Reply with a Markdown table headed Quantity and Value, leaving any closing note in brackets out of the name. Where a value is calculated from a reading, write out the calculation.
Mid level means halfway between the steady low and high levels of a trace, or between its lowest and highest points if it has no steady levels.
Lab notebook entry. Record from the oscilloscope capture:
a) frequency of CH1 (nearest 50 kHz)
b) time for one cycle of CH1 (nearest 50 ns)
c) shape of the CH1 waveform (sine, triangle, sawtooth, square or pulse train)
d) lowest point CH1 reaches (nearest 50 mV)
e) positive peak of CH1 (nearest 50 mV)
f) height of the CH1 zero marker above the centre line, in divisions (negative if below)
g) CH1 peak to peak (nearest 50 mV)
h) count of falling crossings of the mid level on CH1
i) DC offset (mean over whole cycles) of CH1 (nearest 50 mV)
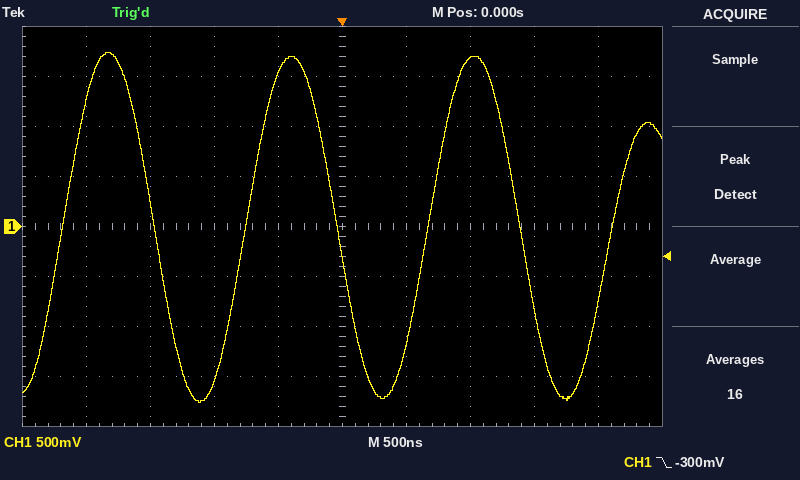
| Quantity | Value |
|---|---|
| frequency of CH1 | 1 / 1.45 µs ≈ 690 kHz, so 700 kHz to the nearest 50 kHz |
| time for one cycle of CH1 | 1.45 µs |
| shape of the CH1 waveform | sine |
| lowest point CH1 reaches | -1.75 V |
| positive peak of CH1 | 1.75 V |
| height of the CH1 zero marker above the centre line, in divisions | 0.0 div |
| CH1 peak to peak | 1.75 V − (-1.75 V) = 3.50 V |
| count of falling crossings of the mid level on CH1 | 3 |
| DC offset (mean over whole cycles) of CH1 | (1.75 V + (-1.75 V)) / 2 ≈ 0 mV |
